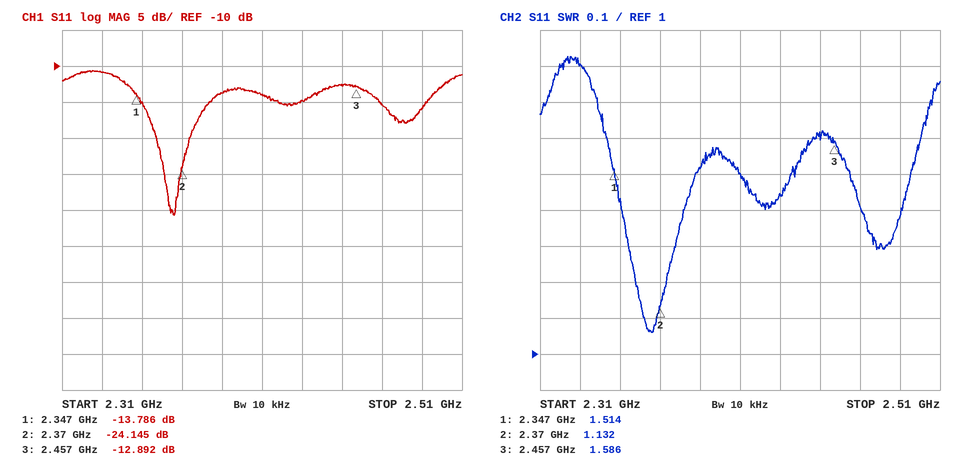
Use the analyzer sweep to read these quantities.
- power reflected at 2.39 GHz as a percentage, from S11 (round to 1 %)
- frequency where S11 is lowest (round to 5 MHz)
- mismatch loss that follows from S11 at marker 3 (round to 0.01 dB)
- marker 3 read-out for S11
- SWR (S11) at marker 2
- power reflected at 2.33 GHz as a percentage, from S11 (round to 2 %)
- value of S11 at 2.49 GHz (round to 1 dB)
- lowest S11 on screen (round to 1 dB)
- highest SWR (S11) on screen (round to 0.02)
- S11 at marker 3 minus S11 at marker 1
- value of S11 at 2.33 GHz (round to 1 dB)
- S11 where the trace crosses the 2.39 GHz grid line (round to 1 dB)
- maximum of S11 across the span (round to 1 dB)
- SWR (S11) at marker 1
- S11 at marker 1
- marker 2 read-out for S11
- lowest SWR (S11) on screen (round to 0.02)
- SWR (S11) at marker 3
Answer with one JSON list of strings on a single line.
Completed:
["4 %", "2.365 GHz", "0.23 dB", "-12.892 dB", "1.132", "8 %", "-16 dB", "-31 dB", "1.82", "0.894 dB", "-11 dB", "-14 dB", "-11 dB", "1.514", "-13.786 dB", "-24.145 dB", "1.06", "1.586"]
